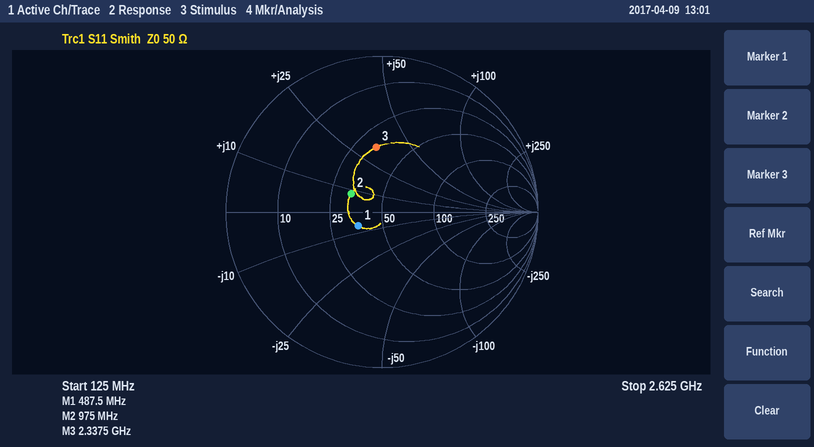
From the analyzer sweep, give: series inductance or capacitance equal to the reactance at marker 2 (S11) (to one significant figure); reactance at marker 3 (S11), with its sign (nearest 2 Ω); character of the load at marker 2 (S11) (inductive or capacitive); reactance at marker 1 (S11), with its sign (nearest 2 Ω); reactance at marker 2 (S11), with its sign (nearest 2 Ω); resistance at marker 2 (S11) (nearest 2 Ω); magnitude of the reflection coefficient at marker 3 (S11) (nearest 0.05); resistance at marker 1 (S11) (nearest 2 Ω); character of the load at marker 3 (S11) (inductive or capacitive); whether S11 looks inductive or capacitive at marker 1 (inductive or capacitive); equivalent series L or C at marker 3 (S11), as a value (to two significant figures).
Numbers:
1 nH
+34 Ω
inductive
-6 Ω
+8 Ω
32 Ω
0.40
36 Ω
inductive
capacitive
2.3 nH
